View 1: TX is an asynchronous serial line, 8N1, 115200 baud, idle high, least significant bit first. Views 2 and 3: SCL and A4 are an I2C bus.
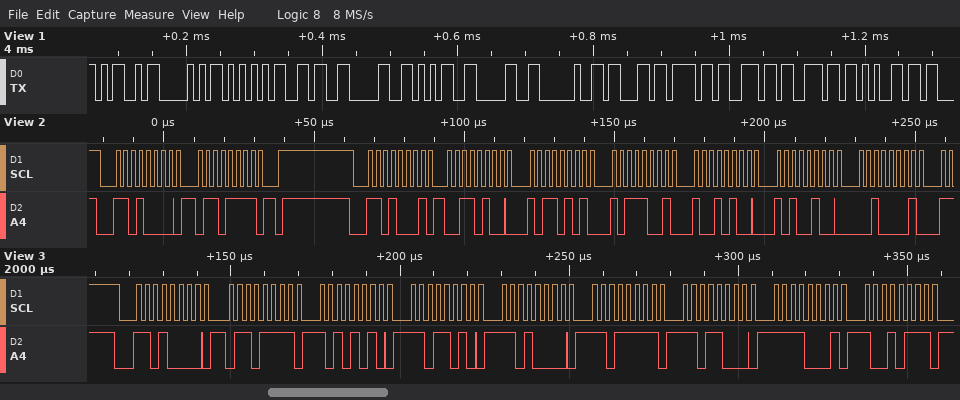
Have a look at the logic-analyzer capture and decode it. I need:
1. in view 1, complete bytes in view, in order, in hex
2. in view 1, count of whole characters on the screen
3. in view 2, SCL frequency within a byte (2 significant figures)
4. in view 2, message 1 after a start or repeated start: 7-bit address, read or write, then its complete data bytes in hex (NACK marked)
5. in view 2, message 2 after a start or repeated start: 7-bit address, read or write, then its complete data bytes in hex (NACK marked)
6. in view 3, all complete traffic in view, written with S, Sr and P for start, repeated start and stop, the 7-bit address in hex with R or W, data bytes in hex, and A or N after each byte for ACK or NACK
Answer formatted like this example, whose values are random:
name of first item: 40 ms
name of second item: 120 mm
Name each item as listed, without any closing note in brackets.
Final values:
in view 1, complete bytes in view, in order, in hex: 4D 50 55 36 30 35 30 20 63 6F 6E 6E 65
in view 1, count of whole characters on the screen: 13
in view 2, SCL frequency within a byte: 400 kHz
in view 2, message 1 after a start or repeated start: 7-bit address, read or write, then its complete data bytes in hex: 0x68 write: 6F
in view 2, message 2 after a start or repeated start: 7-bit address, read or write, then its complete data bytes in hex: 0x68 read: 34 B5 B9 94 A4 21
in view 3, all complete traffic in view, written with S, Sr and P for start, repeated start and stop, the 7-bit address in hex with R or W, data bytes in hex, and A or N after each byte for ACK or NACK: S 68W A 6F A AA A DA A D0 A DF A D8 A F1 A 97 A
